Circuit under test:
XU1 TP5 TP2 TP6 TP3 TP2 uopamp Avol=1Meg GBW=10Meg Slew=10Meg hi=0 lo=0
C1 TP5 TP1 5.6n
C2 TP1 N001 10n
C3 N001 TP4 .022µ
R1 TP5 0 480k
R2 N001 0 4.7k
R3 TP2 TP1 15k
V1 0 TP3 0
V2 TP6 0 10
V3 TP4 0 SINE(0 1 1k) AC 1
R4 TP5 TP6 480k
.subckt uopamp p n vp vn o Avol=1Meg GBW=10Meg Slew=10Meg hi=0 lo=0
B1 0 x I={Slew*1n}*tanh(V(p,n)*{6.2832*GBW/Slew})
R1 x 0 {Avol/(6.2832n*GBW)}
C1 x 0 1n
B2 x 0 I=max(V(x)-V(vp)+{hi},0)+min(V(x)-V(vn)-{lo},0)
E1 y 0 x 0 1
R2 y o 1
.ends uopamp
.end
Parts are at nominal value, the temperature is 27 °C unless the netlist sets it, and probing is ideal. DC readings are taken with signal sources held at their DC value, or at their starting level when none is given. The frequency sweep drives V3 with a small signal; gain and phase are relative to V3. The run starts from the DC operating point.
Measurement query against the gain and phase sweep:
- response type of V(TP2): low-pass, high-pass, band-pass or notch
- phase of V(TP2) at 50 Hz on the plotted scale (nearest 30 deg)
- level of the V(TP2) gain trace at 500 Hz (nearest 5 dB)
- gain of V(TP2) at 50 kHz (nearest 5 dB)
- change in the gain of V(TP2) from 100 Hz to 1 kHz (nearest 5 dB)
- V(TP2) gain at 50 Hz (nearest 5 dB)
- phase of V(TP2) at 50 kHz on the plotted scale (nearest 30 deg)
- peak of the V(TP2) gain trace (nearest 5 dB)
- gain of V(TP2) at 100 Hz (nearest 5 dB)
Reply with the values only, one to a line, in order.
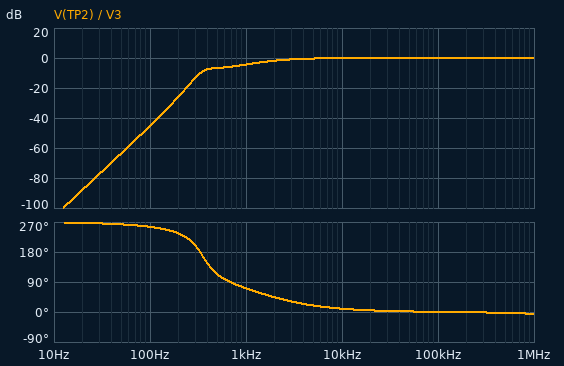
high-pass
270 deg
-5 dB
0 dB
40 dB
-65 dB
0 deg
0 dB
-45 dB
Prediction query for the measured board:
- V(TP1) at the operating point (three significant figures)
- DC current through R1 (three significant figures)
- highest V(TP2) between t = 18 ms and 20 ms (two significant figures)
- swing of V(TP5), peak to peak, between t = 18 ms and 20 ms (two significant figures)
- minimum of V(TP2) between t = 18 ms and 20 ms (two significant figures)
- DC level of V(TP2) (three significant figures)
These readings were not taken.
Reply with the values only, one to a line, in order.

5.00 V
10.4 µA
5.6 V
1.2 V
4.4 V
5.00 V
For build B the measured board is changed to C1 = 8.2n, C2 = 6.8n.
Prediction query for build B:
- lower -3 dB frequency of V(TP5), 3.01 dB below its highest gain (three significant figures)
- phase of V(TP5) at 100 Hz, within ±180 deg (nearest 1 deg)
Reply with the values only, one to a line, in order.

1.39 kHz
-104 deg
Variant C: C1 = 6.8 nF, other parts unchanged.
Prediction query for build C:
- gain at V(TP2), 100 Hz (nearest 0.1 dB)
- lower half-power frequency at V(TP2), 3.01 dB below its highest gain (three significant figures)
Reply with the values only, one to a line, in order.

-43.4 dB
1.42 kHz
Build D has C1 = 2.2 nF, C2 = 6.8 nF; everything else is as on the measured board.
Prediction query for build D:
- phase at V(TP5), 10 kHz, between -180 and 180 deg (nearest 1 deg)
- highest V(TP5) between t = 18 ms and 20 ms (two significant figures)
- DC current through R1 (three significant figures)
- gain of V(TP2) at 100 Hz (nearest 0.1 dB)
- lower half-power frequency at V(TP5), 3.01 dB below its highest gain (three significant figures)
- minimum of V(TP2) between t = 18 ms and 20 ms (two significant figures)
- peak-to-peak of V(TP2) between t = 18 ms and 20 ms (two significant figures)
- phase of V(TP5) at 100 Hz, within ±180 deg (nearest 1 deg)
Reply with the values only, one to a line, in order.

11 deg
5.8 V
10.4 µA
-57.1 dB
788 Hz
4.2 V
1.6 V
-100 deg
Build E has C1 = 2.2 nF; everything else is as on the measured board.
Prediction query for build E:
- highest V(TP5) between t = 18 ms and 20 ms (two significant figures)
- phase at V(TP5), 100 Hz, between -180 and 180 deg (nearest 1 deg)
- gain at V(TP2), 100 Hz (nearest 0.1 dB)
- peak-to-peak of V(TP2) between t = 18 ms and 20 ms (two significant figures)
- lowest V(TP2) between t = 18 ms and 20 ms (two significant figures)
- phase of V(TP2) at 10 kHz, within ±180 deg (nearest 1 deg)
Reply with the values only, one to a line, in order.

5.7 V
-102 deg
-53.7 dB
1.4 V
4.3 V
11 deg
